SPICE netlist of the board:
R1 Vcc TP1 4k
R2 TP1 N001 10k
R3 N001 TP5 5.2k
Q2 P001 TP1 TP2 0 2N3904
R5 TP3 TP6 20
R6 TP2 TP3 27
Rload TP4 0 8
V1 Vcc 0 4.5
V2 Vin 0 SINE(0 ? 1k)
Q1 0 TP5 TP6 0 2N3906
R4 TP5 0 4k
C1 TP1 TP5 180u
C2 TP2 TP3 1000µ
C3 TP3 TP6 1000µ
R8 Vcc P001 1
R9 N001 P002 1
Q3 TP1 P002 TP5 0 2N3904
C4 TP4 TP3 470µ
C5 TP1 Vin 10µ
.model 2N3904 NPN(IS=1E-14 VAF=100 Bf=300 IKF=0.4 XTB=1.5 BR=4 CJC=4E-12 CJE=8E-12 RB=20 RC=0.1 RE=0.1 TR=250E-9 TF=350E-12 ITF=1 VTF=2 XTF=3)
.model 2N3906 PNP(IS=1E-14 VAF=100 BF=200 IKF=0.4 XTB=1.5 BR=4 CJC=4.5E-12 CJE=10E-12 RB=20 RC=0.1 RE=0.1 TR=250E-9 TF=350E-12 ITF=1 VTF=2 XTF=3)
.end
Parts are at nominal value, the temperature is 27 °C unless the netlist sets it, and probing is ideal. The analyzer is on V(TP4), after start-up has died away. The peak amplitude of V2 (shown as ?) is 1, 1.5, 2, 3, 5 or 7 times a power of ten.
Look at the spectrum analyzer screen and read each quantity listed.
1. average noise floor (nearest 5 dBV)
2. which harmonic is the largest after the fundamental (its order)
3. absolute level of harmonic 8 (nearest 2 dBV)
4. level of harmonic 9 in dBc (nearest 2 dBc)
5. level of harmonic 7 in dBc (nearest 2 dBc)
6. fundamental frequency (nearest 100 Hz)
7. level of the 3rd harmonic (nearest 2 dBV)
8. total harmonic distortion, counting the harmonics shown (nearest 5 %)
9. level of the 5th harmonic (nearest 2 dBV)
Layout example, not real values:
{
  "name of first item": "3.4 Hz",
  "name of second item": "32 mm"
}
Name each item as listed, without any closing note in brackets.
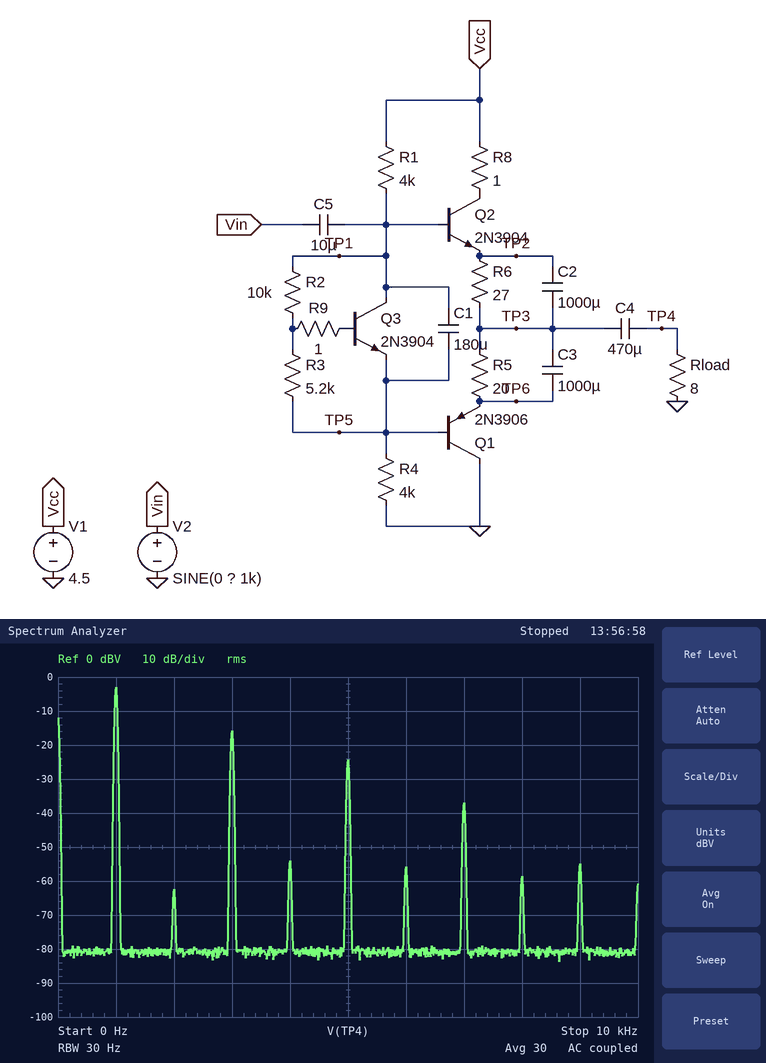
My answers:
{
  "average noise floor": "-80 dBV",
  "which harmonic is the largest after the fundamental": "3",
  "absolute level of harmonic 8": "-58 dBV",
  "level of harmonic 9 in dBc": "-52 dBc",
  "level of harmonic 7 in dBc": "-34 dBc",
  "fundamental frequency": "1.0 kHz",
  "level of the 3rd harmonic": "-16 dBV",
  "total harmonic distortion, counting the harmonics shown": "25 %",
  "level of the 5th harmonic": "-24 dBV"
}
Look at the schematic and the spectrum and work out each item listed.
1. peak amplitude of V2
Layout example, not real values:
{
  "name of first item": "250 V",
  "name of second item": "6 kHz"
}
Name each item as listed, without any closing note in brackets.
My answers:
{
  "peak amplitude of V2": "2 V"
}
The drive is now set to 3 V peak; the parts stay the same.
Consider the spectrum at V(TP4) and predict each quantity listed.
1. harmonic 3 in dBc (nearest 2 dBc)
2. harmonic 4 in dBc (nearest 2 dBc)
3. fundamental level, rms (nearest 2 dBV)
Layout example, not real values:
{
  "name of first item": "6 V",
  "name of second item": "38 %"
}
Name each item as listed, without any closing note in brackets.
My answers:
{
  "harmonic 3 in dBc": "-10 dBc",
  "harmonic 4 in dBc": "-50 dBc",
  "fundamental level, rms": "-2 dBV"
}
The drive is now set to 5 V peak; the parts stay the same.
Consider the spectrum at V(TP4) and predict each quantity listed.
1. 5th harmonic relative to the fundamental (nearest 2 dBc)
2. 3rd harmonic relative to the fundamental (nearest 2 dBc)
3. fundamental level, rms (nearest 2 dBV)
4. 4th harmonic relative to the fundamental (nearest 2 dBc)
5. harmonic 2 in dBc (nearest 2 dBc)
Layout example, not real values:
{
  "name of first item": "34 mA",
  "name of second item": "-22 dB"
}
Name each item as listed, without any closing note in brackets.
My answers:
{
  "5th harmonic relative to the fundamental": "-20 dBc",
  "3rd harmonic relative to the fundamental": "-8 dBc",
  "fundamental level, rms": "-2 dBV",
  "4th harmonic relative to the fundamental": "-58 dBc",
  "harmonic 2 in dBc": "-56 dBc"
}
